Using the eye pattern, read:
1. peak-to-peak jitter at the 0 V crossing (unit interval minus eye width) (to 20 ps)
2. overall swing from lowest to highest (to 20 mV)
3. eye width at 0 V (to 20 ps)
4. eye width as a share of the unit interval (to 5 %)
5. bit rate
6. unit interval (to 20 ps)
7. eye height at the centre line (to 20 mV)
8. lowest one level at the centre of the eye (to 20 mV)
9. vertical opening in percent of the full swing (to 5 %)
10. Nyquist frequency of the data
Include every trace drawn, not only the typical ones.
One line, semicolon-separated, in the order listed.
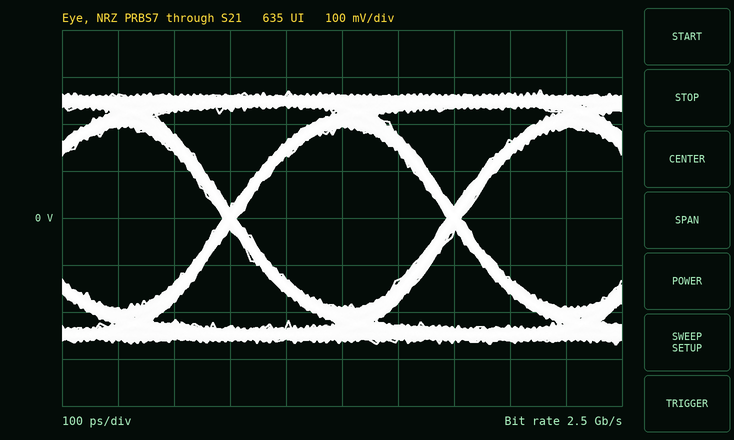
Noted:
20 ps; 540 mV; 380 ps; 95 %; 2.5 Gb/s; 400 ps; 380 mV; 200 mV; 70 %; 1.25 GHz
